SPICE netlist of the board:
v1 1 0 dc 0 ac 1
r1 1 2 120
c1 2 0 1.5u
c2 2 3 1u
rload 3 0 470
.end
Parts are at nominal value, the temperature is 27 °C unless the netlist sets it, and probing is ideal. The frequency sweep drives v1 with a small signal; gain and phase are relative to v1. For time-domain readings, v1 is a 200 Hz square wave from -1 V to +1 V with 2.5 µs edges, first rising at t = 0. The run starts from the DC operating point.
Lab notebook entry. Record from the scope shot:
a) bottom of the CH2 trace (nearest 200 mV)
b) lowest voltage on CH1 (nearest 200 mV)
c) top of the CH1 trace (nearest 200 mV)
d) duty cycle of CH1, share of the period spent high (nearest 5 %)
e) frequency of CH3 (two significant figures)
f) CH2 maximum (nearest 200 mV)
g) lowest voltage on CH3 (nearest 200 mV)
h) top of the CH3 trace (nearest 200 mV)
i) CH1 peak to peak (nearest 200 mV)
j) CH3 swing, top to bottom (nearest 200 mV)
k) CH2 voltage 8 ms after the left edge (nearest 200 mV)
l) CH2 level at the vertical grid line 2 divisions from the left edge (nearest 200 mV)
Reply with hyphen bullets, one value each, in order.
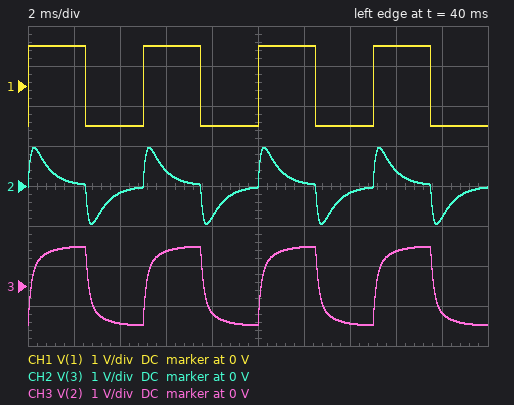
- -1.0 V
- -1.0 V
- 1.0 V
- 50 %
- 200 Hz
- 1.0 V
- -1.0 V
- 1.0 V
- 2.0 V
- 2.0 V
- -800 mV
- -200 mV
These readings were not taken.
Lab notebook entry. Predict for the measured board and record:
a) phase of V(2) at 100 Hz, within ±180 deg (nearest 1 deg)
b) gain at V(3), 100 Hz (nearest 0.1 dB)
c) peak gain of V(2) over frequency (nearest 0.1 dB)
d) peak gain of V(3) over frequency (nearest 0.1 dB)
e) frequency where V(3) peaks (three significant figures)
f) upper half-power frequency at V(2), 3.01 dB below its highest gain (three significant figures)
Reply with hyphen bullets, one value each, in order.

- -10 deg
- -11.3 dB
- 0 dB
- -4.3 dB
- 547 Hz
- 577 Hz
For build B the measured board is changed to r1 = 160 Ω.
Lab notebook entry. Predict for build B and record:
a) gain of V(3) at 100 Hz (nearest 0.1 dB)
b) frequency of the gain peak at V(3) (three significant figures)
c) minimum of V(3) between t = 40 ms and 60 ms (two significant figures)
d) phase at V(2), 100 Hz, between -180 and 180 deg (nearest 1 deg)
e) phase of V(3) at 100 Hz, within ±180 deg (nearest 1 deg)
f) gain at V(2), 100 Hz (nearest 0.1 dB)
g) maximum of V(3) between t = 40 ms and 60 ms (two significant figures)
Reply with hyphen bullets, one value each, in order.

- -11.4 dB
- 474 Hz
- -830 mV
- -13 deg
- 60 deg
- -0.5 dB
- 830 mV
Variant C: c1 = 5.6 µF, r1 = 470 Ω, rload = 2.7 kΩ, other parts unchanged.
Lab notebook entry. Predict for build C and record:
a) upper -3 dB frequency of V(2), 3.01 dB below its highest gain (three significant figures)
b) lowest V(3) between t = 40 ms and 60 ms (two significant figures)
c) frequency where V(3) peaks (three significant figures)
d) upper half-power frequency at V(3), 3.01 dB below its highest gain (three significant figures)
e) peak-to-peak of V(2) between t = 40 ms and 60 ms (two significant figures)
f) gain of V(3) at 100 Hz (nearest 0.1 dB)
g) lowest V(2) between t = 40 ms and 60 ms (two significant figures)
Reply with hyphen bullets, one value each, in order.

- 50.5 Hz
- -370 mV
- 59.7 Hz
- 153 Hz
- 860 mV
- -7.6 dB
- -430 mV
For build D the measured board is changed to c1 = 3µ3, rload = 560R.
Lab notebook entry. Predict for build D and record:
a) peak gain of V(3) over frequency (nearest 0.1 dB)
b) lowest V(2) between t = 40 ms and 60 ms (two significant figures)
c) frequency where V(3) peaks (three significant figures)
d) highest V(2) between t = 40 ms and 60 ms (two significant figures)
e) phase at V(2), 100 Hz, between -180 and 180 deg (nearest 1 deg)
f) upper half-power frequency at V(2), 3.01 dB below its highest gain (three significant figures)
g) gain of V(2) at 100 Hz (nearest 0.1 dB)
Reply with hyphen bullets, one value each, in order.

- -5.7 dB
- -960 mV
- 338 Hz
- 960 mV
- -17 deg
- 307 Hz
- -0.6 dB
